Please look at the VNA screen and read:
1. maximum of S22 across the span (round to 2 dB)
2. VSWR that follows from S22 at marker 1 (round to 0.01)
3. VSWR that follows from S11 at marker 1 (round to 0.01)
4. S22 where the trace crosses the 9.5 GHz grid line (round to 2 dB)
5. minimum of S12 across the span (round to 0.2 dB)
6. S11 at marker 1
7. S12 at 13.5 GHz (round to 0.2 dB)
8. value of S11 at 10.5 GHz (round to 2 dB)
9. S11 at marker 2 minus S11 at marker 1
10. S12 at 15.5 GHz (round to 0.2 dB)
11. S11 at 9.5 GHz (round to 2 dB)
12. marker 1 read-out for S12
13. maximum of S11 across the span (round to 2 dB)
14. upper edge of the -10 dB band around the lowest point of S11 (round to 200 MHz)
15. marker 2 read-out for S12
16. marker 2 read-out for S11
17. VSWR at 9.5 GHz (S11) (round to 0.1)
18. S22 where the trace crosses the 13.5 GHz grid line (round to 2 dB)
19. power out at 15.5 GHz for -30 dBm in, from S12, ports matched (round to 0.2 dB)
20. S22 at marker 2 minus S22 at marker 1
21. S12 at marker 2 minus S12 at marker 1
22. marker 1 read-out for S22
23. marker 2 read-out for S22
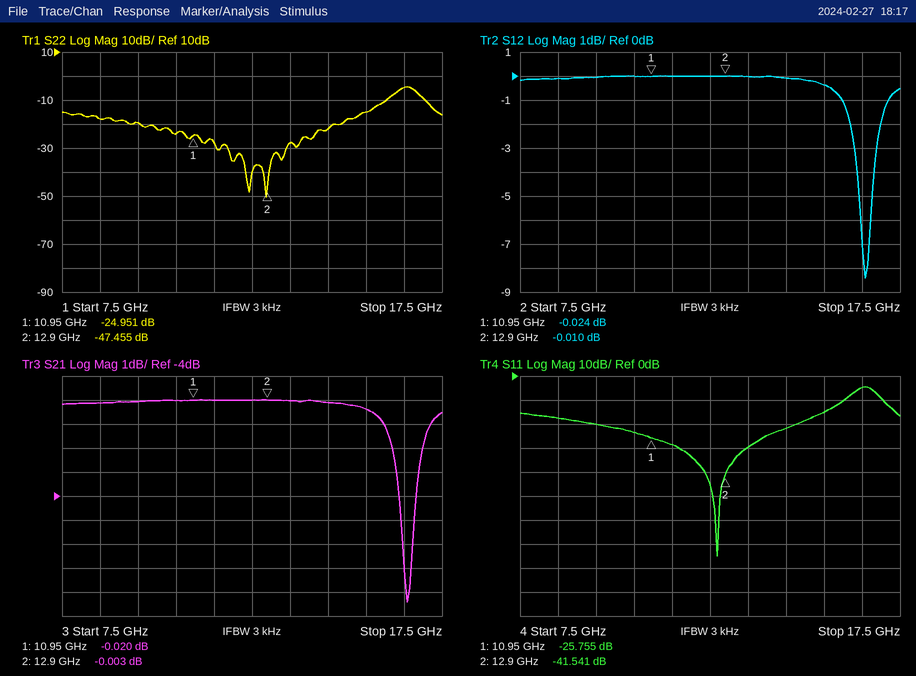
-4 dB
1.12
1.11
-20 dB
-8.4 dB
-25.755 dB
0.0 dB
-24 dB
-15.786 dB
-0.4 dB
-20 dB
-0.024 dB
-4 dB
16.0 GHz
-0.010 dB
-41.541 dB
1.2
-28 dB
-30.4 dBm
-22.504 dB
0.014 dB
-24.951 dB
-47.455 dB
